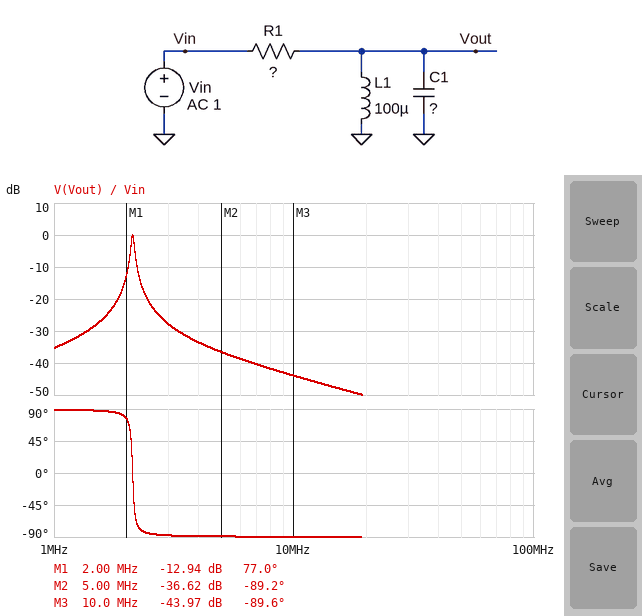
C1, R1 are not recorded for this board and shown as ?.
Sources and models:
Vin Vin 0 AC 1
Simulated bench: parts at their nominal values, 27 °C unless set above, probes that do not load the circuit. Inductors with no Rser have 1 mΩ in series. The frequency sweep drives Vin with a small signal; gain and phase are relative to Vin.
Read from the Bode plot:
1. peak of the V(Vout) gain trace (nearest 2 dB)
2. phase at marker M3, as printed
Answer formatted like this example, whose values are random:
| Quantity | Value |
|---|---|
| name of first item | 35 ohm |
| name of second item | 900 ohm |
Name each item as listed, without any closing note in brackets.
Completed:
| Quantity | Value |
|---|---|
| peak of the V(Vout) gain trace | 0 dB |
| phase at marker M3, as printed | -89.6 deg |
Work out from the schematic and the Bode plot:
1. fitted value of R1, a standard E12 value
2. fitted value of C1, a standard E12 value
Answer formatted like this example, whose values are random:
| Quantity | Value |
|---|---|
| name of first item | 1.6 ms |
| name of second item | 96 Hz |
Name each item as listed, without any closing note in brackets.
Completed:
| Quantity | Value |
|---|---|
| fitted value of R1, a standard E12 value | 47 kΩ |
| fitted value of C1, a standard E12 value | 56 pF |
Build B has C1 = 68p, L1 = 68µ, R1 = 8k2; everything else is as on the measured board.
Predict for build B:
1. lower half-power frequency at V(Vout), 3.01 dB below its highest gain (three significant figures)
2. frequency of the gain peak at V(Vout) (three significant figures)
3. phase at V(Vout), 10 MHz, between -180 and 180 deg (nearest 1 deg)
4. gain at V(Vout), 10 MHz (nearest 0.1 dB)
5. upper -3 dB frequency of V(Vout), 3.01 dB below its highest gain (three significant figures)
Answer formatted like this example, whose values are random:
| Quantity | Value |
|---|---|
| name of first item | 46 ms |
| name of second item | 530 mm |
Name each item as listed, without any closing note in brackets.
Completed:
| Quantity | Value |
|---|---|
| lower half-power frequency at V(Vout), 3.01 dB below its highest gain | 2.20 MHz |
| frequency of the gain peak at V(Vout) | 2.34 MHz |
| phase at V(Vout), 10 MHz, between -180 and 180 deg | -88 deg |
| gain at V(Vout), 10 MHz | -30.4 dB |
| upper -3 dB frequency of V(Vout), 3.01 dB below its highest gain | 2.49 MHz |
